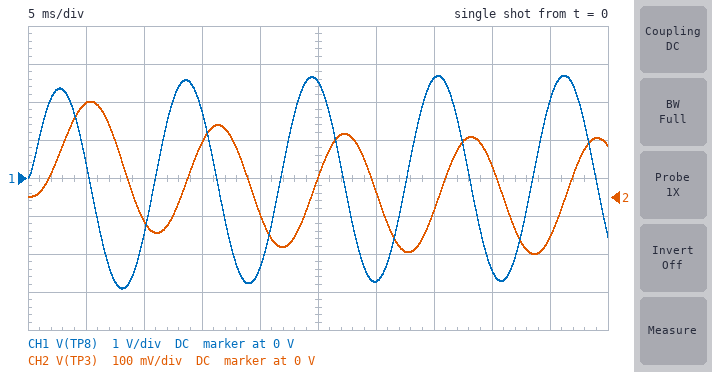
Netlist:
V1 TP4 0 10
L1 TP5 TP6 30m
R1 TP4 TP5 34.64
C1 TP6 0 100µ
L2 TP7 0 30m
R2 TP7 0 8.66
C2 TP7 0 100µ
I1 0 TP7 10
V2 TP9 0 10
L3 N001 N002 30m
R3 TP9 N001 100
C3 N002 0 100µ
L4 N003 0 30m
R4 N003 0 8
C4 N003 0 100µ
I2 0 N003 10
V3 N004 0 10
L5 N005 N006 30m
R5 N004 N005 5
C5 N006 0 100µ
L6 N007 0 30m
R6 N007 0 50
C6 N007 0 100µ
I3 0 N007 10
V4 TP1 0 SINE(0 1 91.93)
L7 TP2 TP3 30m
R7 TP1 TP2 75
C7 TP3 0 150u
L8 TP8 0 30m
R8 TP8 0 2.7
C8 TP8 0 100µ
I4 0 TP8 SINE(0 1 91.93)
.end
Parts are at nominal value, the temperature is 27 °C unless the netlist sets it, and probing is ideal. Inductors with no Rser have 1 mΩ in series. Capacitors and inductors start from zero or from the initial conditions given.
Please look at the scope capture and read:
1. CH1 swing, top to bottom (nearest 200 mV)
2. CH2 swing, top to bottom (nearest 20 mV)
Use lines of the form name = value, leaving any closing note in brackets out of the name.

CH1 swing, top to bottom = 5.6 V
CH2 swing, top to bottom = 400 mV
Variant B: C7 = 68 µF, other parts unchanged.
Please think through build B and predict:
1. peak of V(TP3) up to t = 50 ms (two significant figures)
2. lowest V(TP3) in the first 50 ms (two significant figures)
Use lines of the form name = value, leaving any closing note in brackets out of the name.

peak of V(TP3) up to t = 50 ms = 460 mV
lowest V(TP3) in the first 50 ms = -340 mV
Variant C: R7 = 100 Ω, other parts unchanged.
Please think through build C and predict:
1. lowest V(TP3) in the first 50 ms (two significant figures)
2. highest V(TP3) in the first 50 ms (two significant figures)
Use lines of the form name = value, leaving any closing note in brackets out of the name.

lowest V(TP3) in the first 50 ms = -110 mV
highest V(TP3) in the first 50 ms = 200 mV
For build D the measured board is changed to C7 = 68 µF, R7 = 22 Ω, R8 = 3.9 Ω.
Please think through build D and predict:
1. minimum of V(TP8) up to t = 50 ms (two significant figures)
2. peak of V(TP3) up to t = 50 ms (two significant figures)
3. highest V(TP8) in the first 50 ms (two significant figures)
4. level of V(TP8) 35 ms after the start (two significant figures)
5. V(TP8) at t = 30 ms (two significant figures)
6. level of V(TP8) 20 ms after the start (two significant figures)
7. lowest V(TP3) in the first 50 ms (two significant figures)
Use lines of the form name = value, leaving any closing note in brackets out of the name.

minimum of V(TP8) up to t = 50 ms = -4.2 V
peak of V(TP3) up to t = 50 ms = 1.1 V
highest V(TP8) in the first 50 ms = 3.9 V
level of V(TP8) 35 ms after the start = 3.8 V
V(TP8) at t = 30 ms = -3.9 V
level of V(TP8) 20 ms after the start = -3.4 V
lowest V(TP3) in the first 50 ms = -1.1 V
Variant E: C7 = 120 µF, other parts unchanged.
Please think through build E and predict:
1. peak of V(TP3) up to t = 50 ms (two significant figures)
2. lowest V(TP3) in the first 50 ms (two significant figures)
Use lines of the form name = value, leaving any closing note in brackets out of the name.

peak of V(TP3) up to t = 50 ms = 300 mV
lowest V(TP3) in the first 50 ms = -190 mV
